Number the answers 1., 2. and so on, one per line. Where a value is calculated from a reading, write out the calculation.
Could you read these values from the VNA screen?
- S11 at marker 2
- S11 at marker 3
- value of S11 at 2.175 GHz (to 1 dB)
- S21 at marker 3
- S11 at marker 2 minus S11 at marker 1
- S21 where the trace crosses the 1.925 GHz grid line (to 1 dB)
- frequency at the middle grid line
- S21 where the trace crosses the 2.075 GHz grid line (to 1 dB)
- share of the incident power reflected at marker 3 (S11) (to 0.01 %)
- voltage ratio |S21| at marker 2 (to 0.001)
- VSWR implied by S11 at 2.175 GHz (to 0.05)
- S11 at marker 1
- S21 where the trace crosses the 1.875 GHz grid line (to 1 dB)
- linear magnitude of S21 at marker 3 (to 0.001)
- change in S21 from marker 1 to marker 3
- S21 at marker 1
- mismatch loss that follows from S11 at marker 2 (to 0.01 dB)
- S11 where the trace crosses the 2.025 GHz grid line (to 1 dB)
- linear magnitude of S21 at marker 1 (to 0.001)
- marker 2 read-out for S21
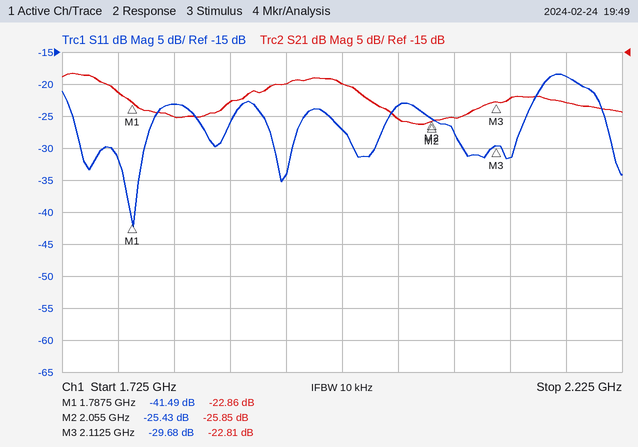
1. -25.43 dB
2. -29.68 dB
3. -19 dB
4. -22.81 dB
5. -25.43 − (-41.49) = 16.06 dB
6. -20 dB
7. 1.975 GHz
8. -25 dB
9. 10^(-29.68/10) ≈ 0.11 %
10. 10^(-25.85/20) ≈ 0.051
11. |Γ| = 10^(-19/20) = 0.1122; VSWR = (1 + 0.1122)/(1 − 0.1122) ≈ 1.25
12. -41.49 dB
13. -23 dB
14. 10^(-22.81/20) ≈ 0.072
15. -22.81 − (-22.86) = 0.05 dB
16. -22.86 dB
17. −10 log10(1 − 10^(-25.43/10)) ≈ 0.01 dB
18. -23 dB
19. 10^(-22.86/20) ≈ 0.072
20. -25.85 dB
